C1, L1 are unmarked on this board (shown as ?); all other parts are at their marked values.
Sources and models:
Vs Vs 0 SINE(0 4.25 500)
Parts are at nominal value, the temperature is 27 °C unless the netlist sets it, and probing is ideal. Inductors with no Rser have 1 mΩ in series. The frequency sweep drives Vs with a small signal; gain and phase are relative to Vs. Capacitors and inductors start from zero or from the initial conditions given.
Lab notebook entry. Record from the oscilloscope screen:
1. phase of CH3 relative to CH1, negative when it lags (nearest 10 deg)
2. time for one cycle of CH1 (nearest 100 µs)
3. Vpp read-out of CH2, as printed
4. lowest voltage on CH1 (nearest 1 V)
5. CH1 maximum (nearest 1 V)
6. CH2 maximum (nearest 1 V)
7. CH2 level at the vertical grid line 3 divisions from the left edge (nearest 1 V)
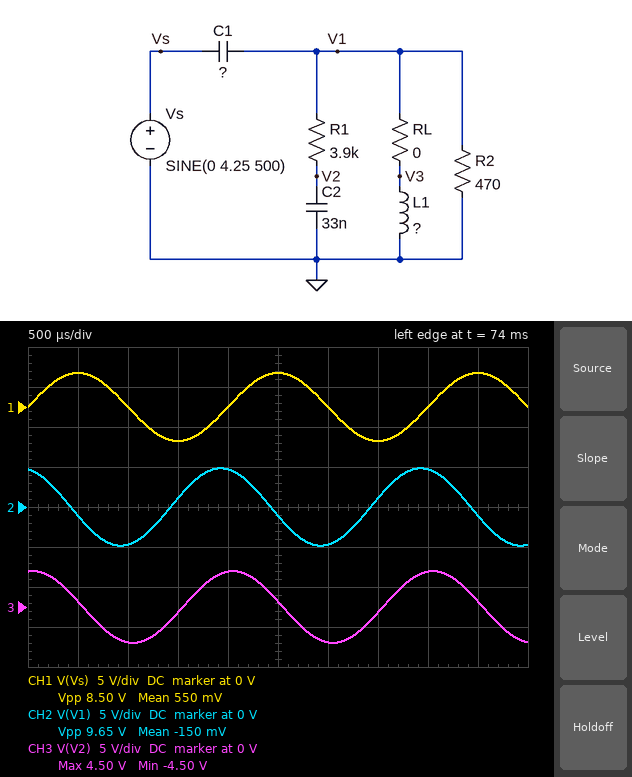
80 deg
2.0 ms
9.65 V
-4 V
4 V
5 V
1 V
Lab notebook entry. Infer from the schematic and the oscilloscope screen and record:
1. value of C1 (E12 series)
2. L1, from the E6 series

820 nF
100 mH
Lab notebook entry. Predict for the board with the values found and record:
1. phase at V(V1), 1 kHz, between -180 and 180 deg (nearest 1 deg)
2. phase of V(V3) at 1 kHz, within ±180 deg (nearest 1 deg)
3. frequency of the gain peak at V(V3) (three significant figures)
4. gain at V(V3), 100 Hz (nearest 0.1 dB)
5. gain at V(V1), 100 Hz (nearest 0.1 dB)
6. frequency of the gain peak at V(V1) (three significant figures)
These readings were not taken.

31 deg
31 deg
622 Hz
-29.6 dB
-29.6 dB
622 Hz
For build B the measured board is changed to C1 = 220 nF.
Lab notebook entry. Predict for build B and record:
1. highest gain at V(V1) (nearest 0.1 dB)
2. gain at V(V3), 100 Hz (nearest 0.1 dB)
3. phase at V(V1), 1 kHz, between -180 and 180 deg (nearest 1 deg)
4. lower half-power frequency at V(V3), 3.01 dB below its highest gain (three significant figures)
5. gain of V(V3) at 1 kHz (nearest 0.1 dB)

0 dB
-41.2 dB
92 deg
1.13 kHz
-4.0 dB
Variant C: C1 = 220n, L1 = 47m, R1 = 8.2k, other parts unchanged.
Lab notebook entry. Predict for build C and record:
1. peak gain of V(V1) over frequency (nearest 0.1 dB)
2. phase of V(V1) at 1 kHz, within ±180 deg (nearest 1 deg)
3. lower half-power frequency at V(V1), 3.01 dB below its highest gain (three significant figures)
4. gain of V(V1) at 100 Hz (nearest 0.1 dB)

1.1 dB
132 deg
1.33 kHz
-47.8 dB
